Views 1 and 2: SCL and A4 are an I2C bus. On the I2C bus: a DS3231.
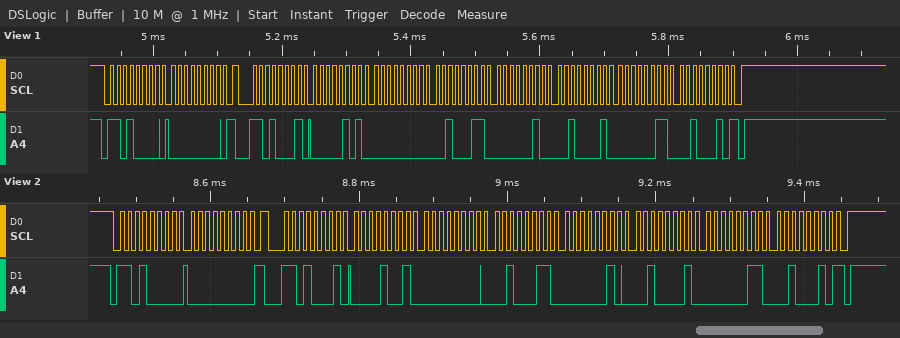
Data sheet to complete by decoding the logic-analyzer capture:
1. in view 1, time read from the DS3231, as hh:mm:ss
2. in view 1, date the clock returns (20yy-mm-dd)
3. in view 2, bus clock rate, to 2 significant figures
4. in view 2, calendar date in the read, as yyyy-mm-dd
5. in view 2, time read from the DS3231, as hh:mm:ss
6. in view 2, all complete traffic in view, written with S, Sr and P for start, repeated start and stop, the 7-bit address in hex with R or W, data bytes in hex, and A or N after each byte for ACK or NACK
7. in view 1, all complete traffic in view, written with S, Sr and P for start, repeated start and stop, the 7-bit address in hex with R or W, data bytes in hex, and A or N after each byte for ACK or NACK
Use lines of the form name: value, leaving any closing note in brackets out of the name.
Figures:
in view 1, time read from the DS3231, as hh:mm:ss: 23:00:05
in view 1, date the clock returns: 2022-03-21
in view 2, bus clock rate, to 2 significant figures: 100 kHz
in view 2, calendar date in the read, as yyyy-mm-dd: 2022-03-21
in view 2, time read from the DS3231, as hh:mm:ss: 23:00:09
in view 2, all complete traffic in view, written with S, Sr and P for start, repeated start and stop, the 7-bit address in hex with R or W, data bytes in hex, and A or N after each byte for ACK or NACK: S 68W A 00 A Sr 68R A 09 A 00 A 23 A 02 A 21 A 03 A 22 N P
in view 1, all complete traffic in view, written with S, Sr and P for start, repeated start and stop, the 7-bit address in hex with R or W, data bytes in hex, and A or N after each byte for ACK or NACK: S 68W A 00 A Sr 68R A 05 A 00 A 23 A 02 A 21 A 03 A 22 N P
